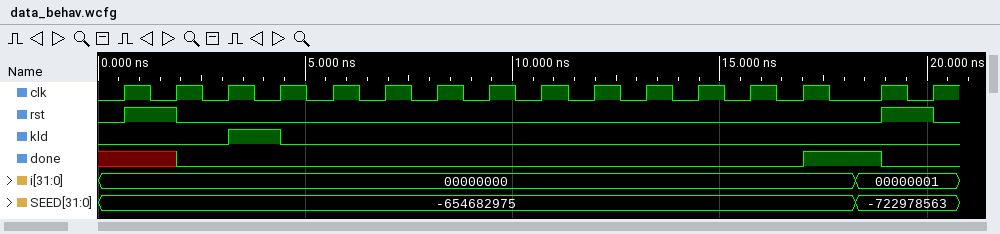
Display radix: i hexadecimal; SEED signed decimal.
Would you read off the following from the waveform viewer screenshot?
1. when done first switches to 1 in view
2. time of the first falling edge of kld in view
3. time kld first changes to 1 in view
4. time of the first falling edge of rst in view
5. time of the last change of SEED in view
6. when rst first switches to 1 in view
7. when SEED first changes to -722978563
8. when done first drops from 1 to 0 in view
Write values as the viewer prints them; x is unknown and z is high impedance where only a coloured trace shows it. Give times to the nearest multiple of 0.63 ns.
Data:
17.01 ns
4.41 ns
3.15 ns
1.89 ns
18.27 ns
0.63 ns
18.27 ns
18.9 ns
